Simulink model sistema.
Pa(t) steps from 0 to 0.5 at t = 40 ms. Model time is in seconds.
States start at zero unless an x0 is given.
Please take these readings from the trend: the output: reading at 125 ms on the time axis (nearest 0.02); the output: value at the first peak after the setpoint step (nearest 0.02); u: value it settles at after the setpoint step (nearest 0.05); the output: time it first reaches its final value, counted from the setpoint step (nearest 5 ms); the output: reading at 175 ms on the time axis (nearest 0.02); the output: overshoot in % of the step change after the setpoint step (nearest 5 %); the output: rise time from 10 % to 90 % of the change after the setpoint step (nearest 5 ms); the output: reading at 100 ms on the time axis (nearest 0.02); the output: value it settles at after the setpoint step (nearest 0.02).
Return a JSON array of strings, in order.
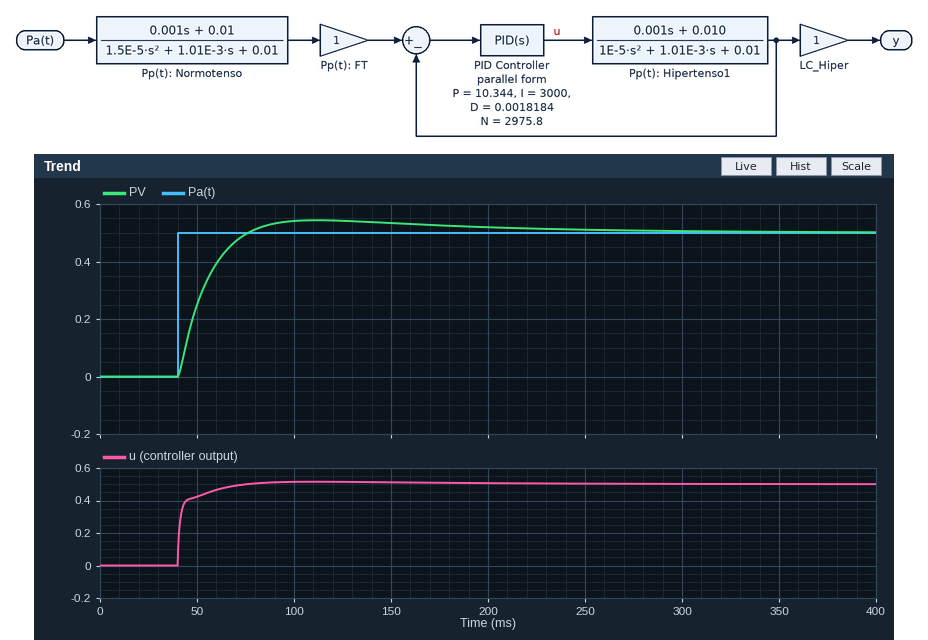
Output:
["0.54", "0.54", "0.50", "35 ms", "0.52", "10 %", "25 ms", "0.54", "0.50"]
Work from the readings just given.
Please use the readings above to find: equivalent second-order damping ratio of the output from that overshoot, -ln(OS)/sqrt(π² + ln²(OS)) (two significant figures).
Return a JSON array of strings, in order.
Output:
["0.59"]
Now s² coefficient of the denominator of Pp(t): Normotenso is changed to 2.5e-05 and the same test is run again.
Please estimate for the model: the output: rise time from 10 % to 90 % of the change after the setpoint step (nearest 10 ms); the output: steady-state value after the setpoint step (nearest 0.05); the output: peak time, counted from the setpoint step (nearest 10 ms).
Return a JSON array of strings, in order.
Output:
["40 ms", "0.50", "100 ms"]
